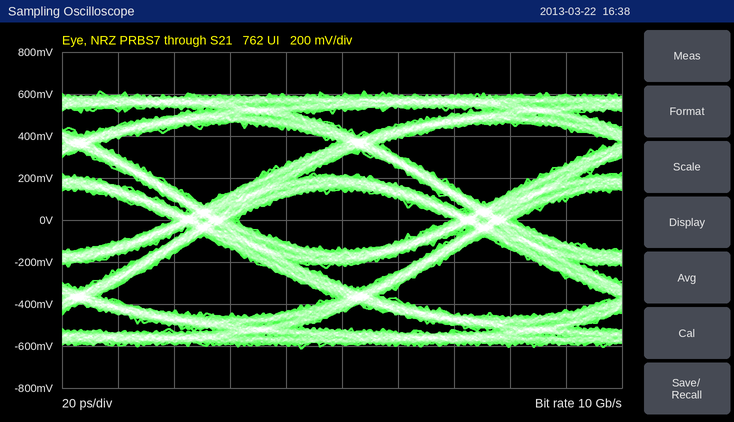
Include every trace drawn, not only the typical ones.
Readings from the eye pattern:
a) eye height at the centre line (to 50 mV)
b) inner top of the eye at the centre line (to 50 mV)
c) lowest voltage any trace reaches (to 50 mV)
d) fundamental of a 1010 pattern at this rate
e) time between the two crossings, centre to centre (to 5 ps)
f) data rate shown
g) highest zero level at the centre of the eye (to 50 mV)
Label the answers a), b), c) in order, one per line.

a) 300 mV
b) 150 mV
c) -600 mV
d) 5 GHz
e) 100 ps
f) 10 Gb/s
g) -150 mV
